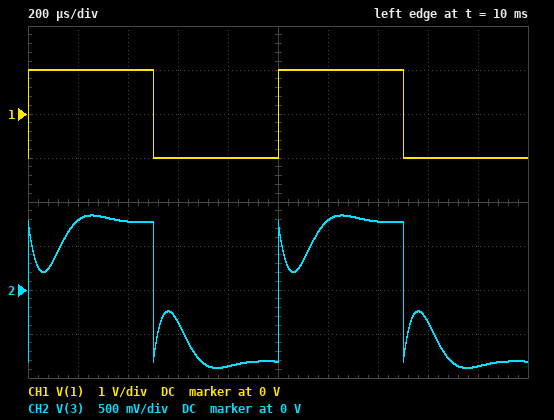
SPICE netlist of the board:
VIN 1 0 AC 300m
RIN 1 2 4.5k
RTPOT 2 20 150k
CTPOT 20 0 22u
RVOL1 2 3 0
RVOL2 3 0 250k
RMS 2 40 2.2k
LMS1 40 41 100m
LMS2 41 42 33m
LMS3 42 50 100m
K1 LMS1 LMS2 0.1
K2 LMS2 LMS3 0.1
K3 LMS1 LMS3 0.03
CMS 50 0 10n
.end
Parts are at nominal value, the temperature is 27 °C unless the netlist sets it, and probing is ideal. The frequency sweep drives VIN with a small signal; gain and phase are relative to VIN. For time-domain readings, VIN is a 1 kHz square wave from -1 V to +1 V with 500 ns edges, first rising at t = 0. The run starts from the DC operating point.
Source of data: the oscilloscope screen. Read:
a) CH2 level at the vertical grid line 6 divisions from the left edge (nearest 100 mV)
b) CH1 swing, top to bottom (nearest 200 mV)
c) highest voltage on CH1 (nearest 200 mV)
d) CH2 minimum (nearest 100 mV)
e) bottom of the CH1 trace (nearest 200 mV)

800 mV
2.0 V
1.0 V
-900 mV
-1.0 V
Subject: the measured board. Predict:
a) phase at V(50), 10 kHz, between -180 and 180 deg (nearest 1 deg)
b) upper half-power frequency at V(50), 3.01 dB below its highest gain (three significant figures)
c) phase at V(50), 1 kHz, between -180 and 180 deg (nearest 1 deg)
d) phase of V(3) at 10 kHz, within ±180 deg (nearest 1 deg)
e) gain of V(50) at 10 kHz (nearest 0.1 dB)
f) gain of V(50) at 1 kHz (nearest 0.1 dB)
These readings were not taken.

-159 deg
3.53 kHz
-22 deg
13 deg
-22.0 dB
-1.7 dB
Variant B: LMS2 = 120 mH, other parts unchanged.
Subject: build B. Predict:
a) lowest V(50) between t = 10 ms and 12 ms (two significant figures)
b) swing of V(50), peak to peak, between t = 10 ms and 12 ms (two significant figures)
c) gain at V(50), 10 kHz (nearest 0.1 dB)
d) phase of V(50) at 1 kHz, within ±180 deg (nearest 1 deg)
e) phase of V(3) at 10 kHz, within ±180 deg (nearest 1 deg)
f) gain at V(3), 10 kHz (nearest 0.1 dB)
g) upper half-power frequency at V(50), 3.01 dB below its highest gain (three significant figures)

-1.1 V
2.2 V
-24.9 dB
-23 deg
9 deg
-2.2 dB
3.08 kHz
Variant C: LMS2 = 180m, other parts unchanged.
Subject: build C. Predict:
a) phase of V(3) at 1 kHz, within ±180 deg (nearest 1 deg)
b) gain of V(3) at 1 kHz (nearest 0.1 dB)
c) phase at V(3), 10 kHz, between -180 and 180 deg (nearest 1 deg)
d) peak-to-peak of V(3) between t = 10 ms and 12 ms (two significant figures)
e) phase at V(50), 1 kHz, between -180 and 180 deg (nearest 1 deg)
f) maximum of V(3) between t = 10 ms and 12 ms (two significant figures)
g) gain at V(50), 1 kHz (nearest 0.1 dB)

-14 deg
-2.6 dB
8 deg
1.8 V
-24 deg
890 mV
-1.1 dB
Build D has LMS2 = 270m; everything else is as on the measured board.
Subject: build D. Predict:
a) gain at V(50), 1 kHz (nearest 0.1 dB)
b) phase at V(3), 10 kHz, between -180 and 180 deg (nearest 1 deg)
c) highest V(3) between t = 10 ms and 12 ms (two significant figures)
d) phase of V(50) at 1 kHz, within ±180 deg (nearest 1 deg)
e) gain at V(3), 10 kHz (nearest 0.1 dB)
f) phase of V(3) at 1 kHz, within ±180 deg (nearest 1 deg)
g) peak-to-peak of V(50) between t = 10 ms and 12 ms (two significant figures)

-0.7 dB
6 deg
900 mV
-25 deg
-2.1 dB
-15 deg
2.4 V
